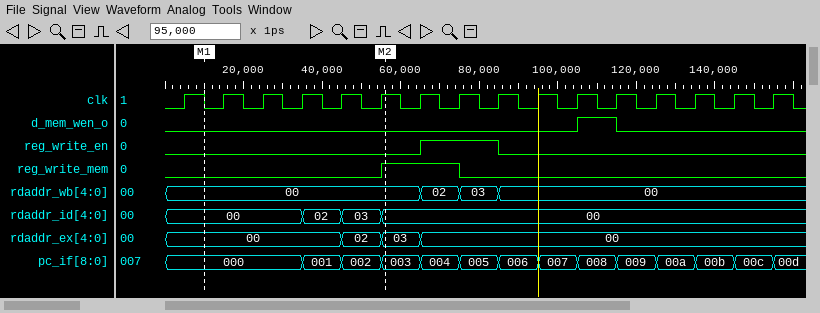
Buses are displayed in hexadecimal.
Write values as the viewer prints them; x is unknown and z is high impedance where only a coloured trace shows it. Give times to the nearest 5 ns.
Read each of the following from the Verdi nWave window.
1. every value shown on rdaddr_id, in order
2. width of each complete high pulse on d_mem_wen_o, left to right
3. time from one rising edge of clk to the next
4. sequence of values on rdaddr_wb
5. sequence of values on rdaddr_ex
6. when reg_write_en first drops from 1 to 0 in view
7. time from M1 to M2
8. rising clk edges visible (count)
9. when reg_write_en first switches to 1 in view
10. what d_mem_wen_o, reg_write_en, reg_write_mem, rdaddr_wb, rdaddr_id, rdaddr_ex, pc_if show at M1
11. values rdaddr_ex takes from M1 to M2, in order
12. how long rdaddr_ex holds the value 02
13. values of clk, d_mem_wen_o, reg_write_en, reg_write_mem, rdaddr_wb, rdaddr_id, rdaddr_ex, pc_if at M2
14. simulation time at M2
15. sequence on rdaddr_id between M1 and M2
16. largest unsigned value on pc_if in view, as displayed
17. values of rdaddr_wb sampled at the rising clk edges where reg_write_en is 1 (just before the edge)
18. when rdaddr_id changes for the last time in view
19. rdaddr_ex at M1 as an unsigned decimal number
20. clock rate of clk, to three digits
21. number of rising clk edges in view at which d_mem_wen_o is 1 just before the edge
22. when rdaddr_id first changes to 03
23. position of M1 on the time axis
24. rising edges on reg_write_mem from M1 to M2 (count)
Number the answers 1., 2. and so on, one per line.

1. 00, 02, 03, 00
2. 10 ns
3. 10 ns
4. 00, 02, 03, 00
5. 00, 02, 03, 00
6. 85 ns
7. 45 ns
8. 16
9. 65 ns
10. d_mem_wen_o=0, reg_write_en=0, reg_write_mem=0, rdaddr_wb=00, rdaddr_id=00, rdaddr_ex=00, pc_if=000
11. 00, 02, 03
12. 10 ns
13. clk=1, d_mem_wen_o=0, reg_write_en=0, reg_write_mem=1, rdaddr_wb=00, rdaddr_id=00, rdaddr_ex=03, pc_if=003
14. 55 ns
15. 00, 02, 03, 00
16. 00d
17. 02, 03
18. 55 ns
19. 0
20. 100 MHz
21. 1
22. 45 ns
23. 10 ns
24. 1
